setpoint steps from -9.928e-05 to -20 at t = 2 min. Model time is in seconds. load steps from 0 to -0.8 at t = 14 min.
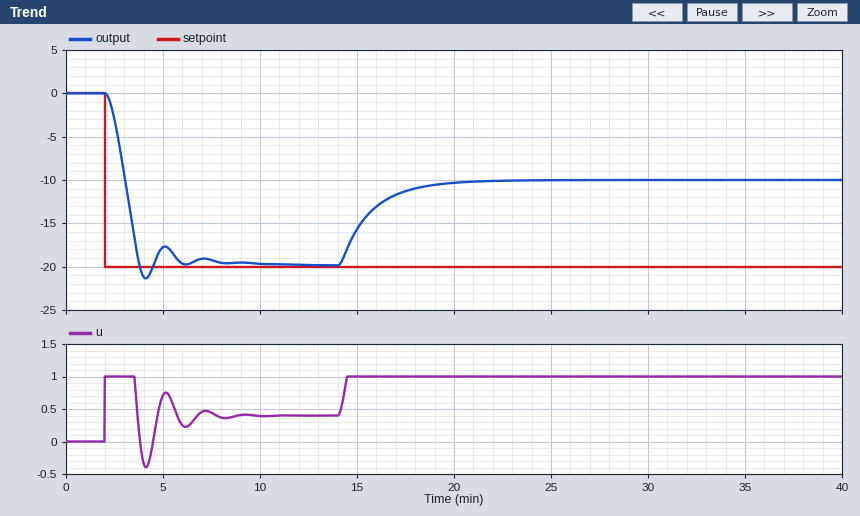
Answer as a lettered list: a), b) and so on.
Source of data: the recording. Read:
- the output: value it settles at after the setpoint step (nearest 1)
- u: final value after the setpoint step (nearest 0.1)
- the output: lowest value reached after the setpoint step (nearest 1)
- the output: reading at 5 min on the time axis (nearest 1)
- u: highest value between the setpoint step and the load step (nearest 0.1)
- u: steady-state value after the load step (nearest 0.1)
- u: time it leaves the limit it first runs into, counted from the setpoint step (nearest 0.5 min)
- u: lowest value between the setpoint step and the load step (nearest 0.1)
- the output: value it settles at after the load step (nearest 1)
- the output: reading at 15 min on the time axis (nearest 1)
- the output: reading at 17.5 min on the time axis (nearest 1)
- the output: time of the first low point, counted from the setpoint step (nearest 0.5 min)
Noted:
a) -20
b) 0.4
c) -21
d) -18
e) 1.0
f) 1.0
g) 1.5 min
h) -0.4
i) -10
j) -16
k) -11
l) 2.0 min
